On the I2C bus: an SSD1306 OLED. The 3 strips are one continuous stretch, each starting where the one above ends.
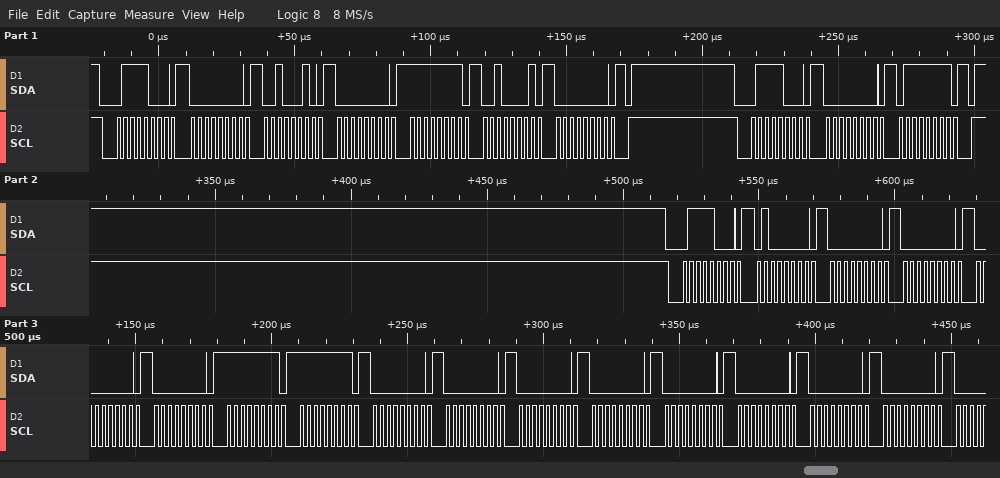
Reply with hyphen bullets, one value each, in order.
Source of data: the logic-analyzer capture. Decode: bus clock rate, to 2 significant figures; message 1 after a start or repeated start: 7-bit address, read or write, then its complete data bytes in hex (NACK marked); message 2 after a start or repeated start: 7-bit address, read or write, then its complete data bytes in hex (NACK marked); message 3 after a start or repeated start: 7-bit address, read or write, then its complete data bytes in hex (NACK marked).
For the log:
- 400 kHz
- 0x3C write: 00 22 00 FF 21 00
- 0x3C write: 00 7F
- 0x3C write: 40 00 00 00 00 FF FF 00 00 00 00 00 00 00 00
